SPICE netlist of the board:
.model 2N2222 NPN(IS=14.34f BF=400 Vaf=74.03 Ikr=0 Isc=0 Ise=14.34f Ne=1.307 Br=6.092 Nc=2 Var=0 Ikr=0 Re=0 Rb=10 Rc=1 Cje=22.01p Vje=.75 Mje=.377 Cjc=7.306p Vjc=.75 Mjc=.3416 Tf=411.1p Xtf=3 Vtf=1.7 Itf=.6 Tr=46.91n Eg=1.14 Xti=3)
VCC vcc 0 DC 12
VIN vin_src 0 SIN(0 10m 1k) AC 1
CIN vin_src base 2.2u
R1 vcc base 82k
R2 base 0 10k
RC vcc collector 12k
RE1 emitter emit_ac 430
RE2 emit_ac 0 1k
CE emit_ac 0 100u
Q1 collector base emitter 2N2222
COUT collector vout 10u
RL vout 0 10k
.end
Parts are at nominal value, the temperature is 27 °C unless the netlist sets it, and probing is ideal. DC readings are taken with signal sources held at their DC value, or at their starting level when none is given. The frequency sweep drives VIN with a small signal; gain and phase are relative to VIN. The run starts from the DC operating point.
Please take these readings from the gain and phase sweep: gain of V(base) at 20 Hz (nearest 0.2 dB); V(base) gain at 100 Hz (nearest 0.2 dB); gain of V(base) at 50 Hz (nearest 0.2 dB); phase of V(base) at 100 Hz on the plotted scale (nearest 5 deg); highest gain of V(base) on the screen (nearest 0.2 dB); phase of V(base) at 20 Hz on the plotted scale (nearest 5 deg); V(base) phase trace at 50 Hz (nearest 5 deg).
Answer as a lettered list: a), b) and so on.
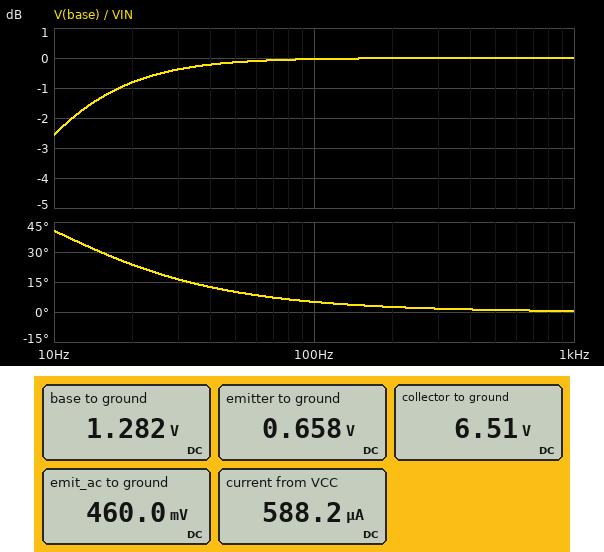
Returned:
a) -0.8 dB
b) 0 dB
c) -0.2 dB
d) 5 deg
e) 0 dB
f) 25 deg
g) 10 deg
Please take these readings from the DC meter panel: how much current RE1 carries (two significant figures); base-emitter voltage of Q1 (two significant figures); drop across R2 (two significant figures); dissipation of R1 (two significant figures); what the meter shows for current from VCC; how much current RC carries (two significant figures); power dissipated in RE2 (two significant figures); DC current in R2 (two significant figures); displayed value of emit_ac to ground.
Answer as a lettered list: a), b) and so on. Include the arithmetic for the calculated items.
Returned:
a) (658 mV - 460 mV) / 430 Ω = 460 µA
b) 1.282 V - 658 mV = 620 mV
c) 1.282 V = 1.3 V
d) (12 V - 1.282 V)^2 / 82 kΩ = 1.4 mW
e) 588.2 µA
f) (12 V - 6.51 V) / 12 kΩ = 460 µA
g) (460 mV)^2 / 1 kΩ = 210 µW
h) (1.282 V) / 10 kΩ = 130 µA
i) 460.0 mV
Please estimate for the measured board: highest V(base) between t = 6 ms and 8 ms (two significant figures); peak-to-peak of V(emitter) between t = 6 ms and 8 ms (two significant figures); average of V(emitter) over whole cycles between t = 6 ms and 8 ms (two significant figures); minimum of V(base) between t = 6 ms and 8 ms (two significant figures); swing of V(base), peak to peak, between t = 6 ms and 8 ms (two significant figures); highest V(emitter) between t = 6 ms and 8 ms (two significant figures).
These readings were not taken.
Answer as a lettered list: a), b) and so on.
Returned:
a) 1.3 V
b) 18 mV
c) 660 mV
d) 1.3 V
e) 20 mV
f) 670 mV
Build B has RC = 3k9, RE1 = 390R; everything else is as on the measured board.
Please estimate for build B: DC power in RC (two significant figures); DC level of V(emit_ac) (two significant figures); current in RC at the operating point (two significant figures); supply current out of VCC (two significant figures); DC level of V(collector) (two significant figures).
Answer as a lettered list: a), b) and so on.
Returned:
a) 870 µW
b) 470 mV
c) 470 µA
d) 600 µA
e) 10 V
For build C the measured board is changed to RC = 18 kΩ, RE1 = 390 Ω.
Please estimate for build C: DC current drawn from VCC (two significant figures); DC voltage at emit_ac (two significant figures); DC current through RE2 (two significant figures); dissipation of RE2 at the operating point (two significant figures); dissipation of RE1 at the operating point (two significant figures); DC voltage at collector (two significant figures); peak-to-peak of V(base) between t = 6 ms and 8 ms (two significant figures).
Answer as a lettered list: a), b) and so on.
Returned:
a) 600 µA
b) 470 mV
c) 470 µA
d) 220 µW
e) 87 µW
f) 3.6 V
g) 20 mV
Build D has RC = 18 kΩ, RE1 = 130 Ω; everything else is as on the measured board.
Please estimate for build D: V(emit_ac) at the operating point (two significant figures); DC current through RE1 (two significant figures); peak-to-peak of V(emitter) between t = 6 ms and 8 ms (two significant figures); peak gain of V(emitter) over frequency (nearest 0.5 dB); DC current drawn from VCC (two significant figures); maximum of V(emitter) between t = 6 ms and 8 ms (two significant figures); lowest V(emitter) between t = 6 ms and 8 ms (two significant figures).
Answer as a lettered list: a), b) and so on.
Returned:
a) 570 mV
b) 570 µA
c) 15 mV
d) -2.5 dB
e) 700 µA
f) 650 mV
g) 640 mV
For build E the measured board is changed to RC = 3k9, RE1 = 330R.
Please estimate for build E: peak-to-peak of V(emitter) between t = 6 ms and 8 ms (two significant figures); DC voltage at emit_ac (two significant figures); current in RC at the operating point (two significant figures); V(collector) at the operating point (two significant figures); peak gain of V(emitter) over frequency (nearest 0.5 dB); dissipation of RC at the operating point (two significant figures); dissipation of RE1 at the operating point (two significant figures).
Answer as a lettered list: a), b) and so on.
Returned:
a) 17 mV
b) 490 mV
c) 490 µA
d) 10 V
e) -1.5 dB
f) 940 µW
g) 80 µW
